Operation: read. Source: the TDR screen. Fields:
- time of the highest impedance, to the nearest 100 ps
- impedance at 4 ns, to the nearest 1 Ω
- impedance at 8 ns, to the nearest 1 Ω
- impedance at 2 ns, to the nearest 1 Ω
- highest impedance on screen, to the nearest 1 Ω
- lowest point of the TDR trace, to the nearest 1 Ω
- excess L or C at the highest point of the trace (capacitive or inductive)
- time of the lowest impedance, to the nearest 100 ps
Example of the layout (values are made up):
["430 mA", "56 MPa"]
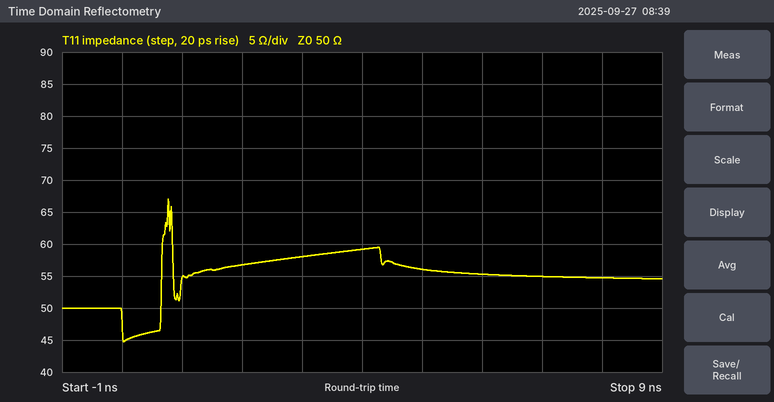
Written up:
["800 ps", "59 Ω", "55 Ω", "57 Ω", "67 Ω", "45 Ω", "inductive", "0.0 ns"]
